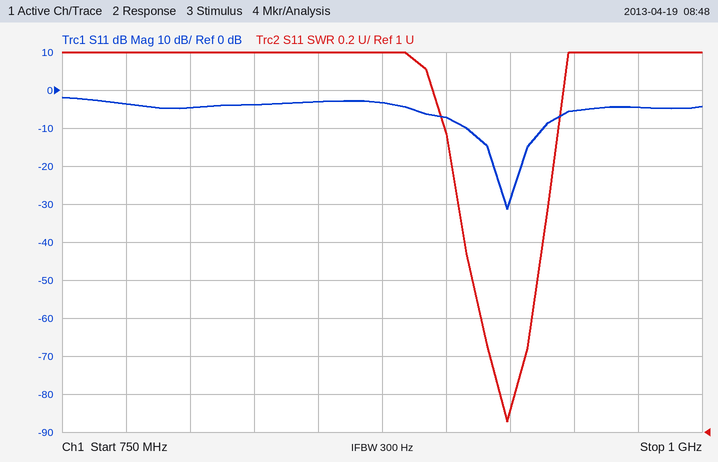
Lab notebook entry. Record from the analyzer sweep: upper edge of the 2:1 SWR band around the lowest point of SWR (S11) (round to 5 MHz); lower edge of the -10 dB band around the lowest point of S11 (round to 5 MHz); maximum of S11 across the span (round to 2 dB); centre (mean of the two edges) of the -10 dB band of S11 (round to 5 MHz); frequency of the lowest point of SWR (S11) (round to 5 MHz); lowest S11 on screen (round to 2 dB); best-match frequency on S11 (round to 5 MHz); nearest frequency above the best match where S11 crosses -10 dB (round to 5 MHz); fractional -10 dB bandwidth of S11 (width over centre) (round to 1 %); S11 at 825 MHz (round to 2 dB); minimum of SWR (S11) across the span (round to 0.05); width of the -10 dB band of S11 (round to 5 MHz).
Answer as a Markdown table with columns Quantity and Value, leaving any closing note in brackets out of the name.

| Quantity | Value |
|---|---|
| upper edge of the 2:1 SWR band around the lowest point of SWR (S11) | 940 MHz |
| lower edge of the -10 dB band around the lowest point of S11 | 910 MHz |
| maximum of S11 across the span | -2 dB |
| centre (mean of the two edges) of the -10 dB band of S11 | 925 MHz |
| frequency of the lowest point of SWR (S11) | 925 MHz |
| lowest S11 on screen | -32 dB |
| best-match frequency on S11 | 925 MHz |
| nearest frequency above the best match where S11 crosses -10 dB | 940 MHz |
| fractional -10 dB bandwidth of S11 (width over centre) | 3 % |
| S11 at 825 MHz | -4 dB |
| minimum of SWR (S11) across the span | 1.05 |
| width of the -10 dB band of S11 | 30 MHz |
